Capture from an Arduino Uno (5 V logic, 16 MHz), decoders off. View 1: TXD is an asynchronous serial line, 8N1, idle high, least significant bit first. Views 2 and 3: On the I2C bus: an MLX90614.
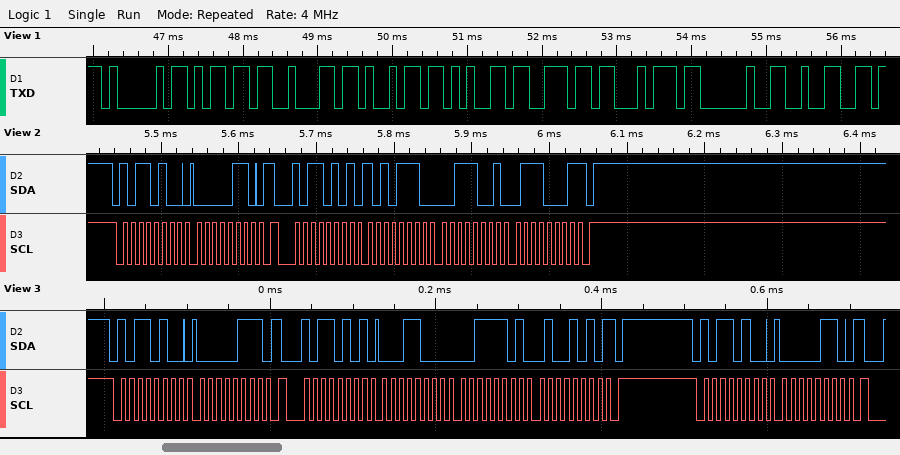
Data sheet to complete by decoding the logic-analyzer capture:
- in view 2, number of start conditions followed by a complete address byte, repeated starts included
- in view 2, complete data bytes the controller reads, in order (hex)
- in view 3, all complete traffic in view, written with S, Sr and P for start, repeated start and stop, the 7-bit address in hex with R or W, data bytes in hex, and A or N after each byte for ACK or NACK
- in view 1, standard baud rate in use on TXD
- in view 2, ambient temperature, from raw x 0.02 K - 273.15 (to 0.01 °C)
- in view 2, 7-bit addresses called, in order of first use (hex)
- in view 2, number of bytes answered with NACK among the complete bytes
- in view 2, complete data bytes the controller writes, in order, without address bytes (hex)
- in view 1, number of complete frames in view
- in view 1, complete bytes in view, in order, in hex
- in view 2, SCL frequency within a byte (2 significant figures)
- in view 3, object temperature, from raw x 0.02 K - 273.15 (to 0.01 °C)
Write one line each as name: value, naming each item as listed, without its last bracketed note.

in view 2, number of start conditions followed by a complete address byte, repeated starts included: 2
in view 2, complete data bytes the controller reads, in order: AE 39 71
in view 3, all complete traffic in view, written with S, Sr and P for start, repeated start and stop, the 7-bit address in hex with R or W, data bytes in hex, and A or N after each byte for ACK or NACK: S 5AW A 07 A Sr 5AR A 18 A 3D A 4A N P S 5AW A 06 A
in view 1, standard baud rate in use on TXD: 9600 baud
in view 2, ambient temperature, from raw x 0.02 K - 273.15: 22.17 °C
in view 2, 7-bit addresses called, in order of first use: 0x5A
in view 2, number of bytes answered with NACK among the complete bytes: 1
in view 2, complete data bytes the controller writes, in order, without address bytes: 06
in view 1, number of complete frames in view: 9
in view 1, complete bytes in view, in order, in hex: 41 6D 62 69 65 6E 74 20 32
in view 2, SCL frequency within a byte: 100 kHz
in view 3, object temperature, from raw x 0.02 K - 273.15: 39.65 °C
